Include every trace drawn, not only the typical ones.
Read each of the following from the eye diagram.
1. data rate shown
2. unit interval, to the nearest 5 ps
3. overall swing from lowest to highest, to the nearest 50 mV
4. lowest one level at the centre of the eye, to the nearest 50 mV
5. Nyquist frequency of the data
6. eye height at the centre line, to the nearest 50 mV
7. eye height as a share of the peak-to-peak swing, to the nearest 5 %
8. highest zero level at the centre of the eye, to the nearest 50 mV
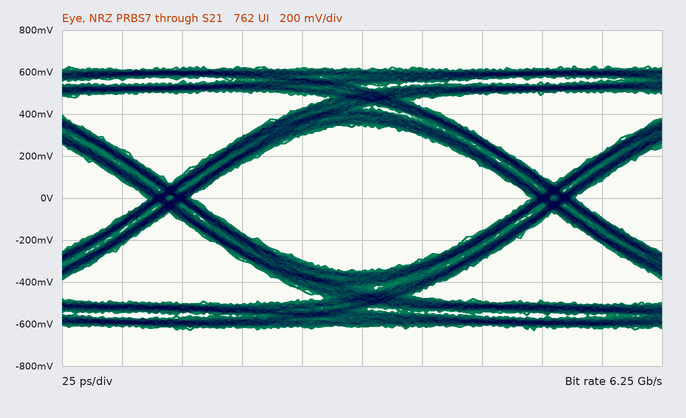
6.25 Gb/s
160 ps
1.25 V
350 mV
3.125 GHz
700 mV
55 %
-350 mV
